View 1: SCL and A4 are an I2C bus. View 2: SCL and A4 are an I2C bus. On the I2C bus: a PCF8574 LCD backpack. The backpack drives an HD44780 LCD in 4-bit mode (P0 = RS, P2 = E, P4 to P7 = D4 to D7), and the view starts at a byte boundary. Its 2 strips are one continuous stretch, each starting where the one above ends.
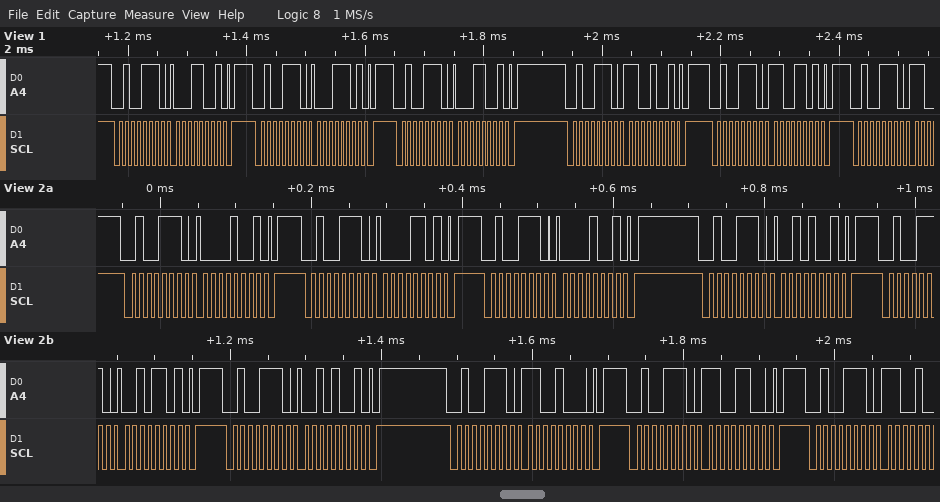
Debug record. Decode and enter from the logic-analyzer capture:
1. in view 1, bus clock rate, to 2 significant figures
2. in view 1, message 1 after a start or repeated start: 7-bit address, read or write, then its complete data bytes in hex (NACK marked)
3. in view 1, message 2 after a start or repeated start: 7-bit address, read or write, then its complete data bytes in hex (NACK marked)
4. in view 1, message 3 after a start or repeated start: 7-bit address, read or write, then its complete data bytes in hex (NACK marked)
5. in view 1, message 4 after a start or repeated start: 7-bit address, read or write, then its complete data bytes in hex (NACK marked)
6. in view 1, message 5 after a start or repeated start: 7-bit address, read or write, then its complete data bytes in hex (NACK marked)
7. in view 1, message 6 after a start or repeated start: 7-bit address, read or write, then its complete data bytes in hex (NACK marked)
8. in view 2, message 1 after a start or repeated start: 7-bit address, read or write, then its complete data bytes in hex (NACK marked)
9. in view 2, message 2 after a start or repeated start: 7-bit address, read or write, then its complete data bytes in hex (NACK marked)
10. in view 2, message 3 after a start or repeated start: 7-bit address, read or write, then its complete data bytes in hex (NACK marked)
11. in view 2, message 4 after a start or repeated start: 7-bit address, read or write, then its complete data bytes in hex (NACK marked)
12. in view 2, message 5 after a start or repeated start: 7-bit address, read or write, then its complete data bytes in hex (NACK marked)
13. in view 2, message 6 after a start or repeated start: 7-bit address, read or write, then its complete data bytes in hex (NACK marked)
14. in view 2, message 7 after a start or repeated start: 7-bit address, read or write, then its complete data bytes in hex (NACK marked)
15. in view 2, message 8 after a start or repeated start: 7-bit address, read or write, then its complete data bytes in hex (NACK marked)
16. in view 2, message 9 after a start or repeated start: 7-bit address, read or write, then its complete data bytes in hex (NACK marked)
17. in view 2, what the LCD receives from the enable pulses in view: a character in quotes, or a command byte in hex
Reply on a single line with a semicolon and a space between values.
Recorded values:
100 kHz; 0x27 write: 19; 0x27 write: 1D; 0x27 write: 19; 0x27 write: C9; 0x27 write: CD; 0x27 write; 0x27 write: 09; 0x27 write: 0D; 0x27 write: 09; 0x27 write: 29; 0x27 write: 2D; 0x27 write: 29; 0x27 write: C8; 0x27 write: CC; 0x27 write; data 0x02
